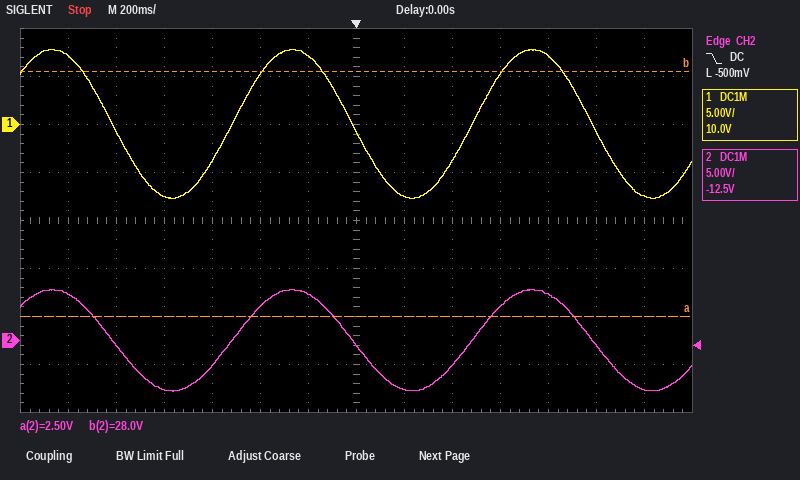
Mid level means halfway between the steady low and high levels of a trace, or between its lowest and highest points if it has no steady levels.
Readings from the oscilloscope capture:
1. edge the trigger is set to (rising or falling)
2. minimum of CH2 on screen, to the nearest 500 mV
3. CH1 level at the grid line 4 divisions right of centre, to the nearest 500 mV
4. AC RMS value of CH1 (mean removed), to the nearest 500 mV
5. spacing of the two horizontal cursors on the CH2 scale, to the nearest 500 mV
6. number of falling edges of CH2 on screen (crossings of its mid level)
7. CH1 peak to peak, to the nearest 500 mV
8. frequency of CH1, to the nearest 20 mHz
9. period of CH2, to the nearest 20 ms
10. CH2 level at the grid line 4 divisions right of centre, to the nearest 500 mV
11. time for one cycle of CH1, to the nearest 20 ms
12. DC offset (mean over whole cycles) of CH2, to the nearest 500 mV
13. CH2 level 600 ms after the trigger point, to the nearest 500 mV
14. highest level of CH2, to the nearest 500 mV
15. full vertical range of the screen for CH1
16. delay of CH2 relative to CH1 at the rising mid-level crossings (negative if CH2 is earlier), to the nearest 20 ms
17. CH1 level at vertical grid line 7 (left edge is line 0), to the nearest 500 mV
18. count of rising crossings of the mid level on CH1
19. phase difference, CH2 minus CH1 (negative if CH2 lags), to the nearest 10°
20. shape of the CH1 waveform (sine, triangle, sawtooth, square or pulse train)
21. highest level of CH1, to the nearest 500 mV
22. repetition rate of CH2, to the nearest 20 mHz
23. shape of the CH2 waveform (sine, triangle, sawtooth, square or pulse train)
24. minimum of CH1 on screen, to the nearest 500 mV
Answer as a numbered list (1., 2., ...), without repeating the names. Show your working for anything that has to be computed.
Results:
1. falling
2. -5.5 V
3. 7.0 V
4. 15.5 V / (2√2) ≈ 5.5 V
5. 25.5 V
6. 3
7. 8.0 V − (-7.5 V) = 15.5 V
8. 1 / 1.00 s ≈ 1.00 Hz
9. 1.00 s
10. 5.0 V
11. 1.00 s
12. (5.5 V + (-5.5 V)) / 2 ≈ 0.0 V
13. 3.5 V
14. 5.5 V
15. 40 V
16. 0 ms
17. -500 mV
18. 2
19. −360° × (0 ms) / 1.00 s ≈ 0°
20. sine
21. 8.0 V
22. 1 / 1.00 s ≈ 1.00 Hz
23. sine
24. -7.5 V
